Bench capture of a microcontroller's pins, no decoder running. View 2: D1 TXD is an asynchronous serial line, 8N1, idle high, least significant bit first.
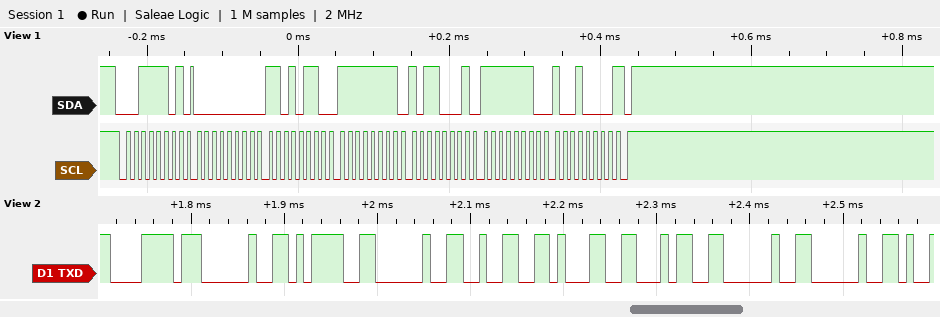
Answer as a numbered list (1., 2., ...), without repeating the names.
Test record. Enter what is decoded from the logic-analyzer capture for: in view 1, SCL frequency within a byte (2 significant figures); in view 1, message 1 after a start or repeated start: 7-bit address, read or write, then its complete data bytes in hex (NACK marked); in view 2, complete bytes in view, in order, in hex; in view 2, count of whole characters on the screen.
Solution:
1. 100 kHz
2. 0x1E read: 00 D6 FF B1 FE 90 NACK
3. 78 20 3D 20 32 31 34 20 20
4. 9
